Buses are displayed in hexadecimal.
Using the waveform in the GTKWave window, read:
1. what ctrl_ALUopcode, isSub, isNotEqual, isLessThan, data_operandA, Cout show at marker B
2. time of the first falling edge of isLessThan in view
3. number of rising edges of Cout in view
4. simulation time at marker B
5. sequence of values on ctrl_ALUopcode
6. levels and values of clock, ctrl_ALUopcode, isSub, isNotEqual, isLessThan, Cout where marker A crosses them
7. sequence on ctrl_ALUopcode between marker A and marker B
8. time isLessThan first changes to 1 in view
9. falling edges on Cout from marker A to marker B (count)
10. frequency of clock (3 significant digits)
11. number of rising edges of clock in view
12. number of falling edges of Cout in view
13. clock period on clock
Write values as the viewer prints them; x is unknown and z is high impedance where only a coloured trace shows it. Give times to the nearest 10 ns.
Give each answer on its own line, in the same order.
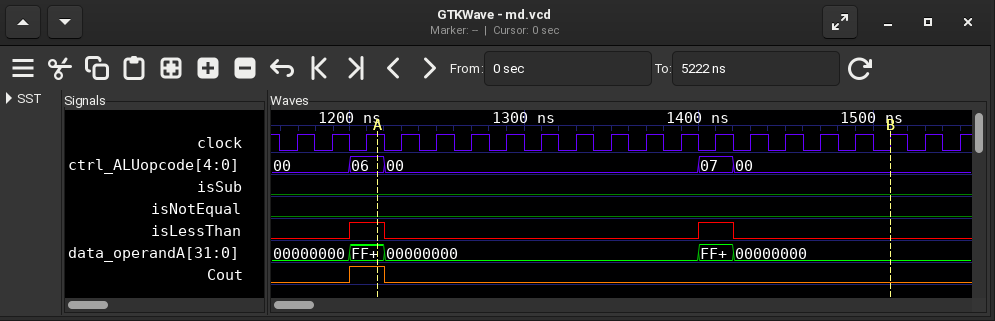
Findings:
ctrl_ALUopcode=00, isSub=0, isNotEqual=0, isLessThan=0, data_operandA=00000000, Cout=0
1220 ns
1
1510 ns
00, 06, 00, 07, 00
clock=1, ctrl_ALUopcode=06, isSub=0, isNotEqual=0, isLessThan=1, Cout=1
06, 00, 07, 00
1200 ns
1
50.0 MHz
20
1
20 ns
